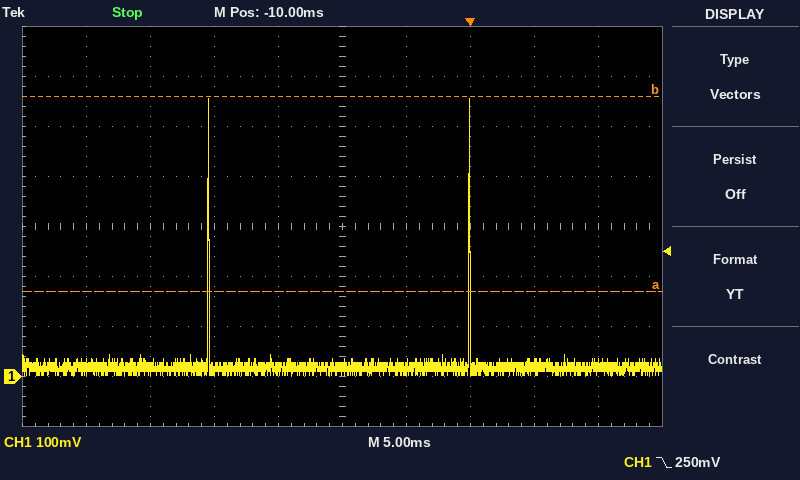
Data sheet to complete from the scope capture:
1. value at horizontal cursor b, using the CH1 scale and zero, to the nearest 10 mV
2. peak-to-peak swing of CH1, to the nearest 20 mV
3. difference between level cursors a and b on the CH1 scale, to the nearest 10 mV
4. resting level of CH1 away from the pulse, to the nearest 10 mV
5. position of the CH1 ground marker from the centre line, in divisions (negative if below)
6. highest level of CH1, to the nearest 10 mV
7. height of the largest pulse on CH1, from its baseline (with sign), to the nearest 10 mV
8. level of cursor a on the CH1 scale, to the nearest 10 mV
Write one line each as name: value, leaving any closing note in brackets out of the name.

value at horizontal cursor b, using the CH1 scale and zero, to the nearest 10 mV: 560 mV
peak-to-peak swing of CH1, to the nearest 20 mV: 560 mV
difference between level cursors a and b on the CH1 scale, to the nearest 10 mV: 390 mV
resting level of CH1 away from the pulse, to the nearest 10 mV: 20 mV
position of the CH1 ground marker from the centre line, in divisions: -3.0 div
highest level of CH1, to the nearest 10 mV: 560 mV
height of the largest pulse on CH1, from its baseline (with sign), to the nearest 10 mV: +540 mV
level of cursor a on the CH1 scale, to the nearest 10 mV: 170 mV
